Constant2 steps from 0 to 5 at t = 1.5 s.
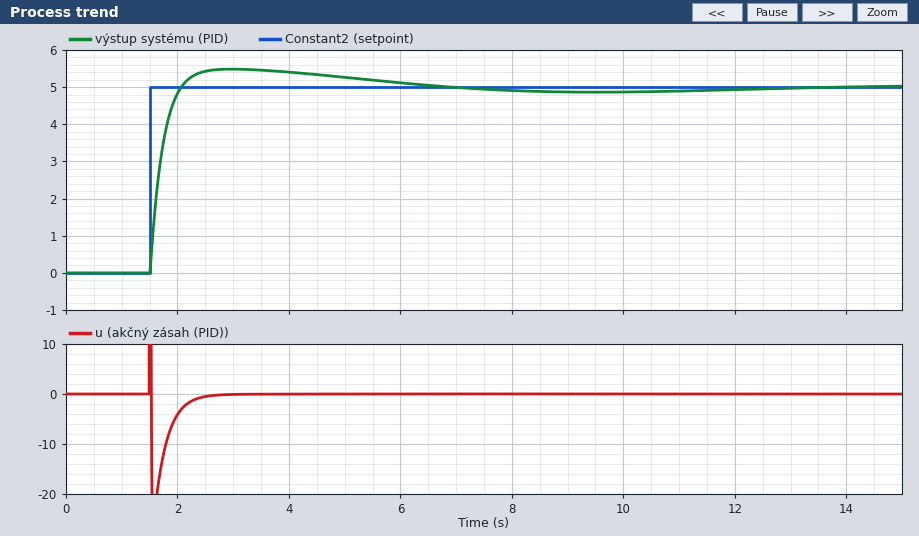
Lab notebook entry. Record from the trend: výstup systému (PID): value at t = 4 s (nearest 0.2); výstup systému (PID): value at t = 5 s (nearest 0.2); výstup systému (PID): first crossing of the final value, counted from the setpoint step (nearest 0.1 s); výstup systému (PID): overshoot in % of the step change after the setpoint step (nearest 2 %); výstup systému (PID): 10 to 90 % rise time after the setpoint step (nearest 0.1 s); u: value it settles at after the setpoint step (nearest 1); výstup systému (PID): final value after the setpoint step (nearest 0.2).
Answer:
5.4
5.2
0.6 s
10 %
0.4 s
0
5.0
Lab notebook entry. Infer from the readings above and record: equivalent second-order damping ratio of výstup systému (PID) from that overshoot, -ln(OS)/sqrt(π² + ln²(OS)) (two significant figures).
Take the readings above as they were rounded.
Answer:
0.59
